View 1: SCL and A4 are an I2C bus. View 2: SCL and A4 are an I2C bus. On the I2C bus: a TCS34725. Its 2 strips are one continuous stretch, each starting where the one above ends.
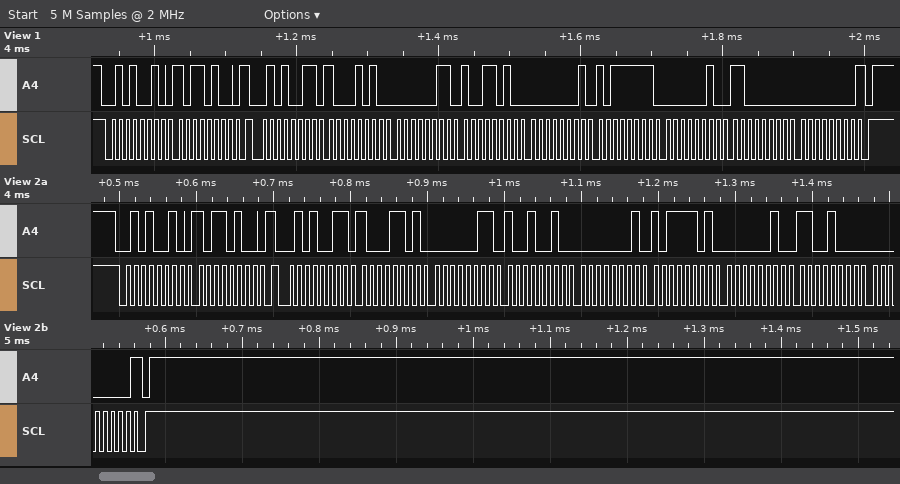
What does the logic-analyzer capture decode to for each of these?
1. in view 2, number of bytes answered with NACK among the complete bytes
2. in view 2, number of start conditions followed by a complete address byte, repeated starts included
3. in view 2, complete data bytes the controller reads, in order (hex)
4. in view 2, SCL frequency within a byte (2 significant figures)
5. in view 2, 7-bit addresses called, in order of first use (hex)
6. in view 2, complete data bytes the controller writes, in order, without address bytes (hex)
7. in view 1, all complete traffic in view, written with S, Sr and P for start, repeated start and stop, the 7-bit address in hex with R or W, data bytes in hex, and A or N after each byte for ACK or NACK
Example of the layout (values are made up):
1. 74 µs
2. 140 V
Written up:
1. 1
2. 2
3. 8D 03 92 01 BD 02 C8 00
4. 100 kHz
5. 0x29
6. B4
7. S 29W A B4 A Sr 29R A 8A A 03 A 9A A 01 A BF A 02 A C0 A 00 N P
